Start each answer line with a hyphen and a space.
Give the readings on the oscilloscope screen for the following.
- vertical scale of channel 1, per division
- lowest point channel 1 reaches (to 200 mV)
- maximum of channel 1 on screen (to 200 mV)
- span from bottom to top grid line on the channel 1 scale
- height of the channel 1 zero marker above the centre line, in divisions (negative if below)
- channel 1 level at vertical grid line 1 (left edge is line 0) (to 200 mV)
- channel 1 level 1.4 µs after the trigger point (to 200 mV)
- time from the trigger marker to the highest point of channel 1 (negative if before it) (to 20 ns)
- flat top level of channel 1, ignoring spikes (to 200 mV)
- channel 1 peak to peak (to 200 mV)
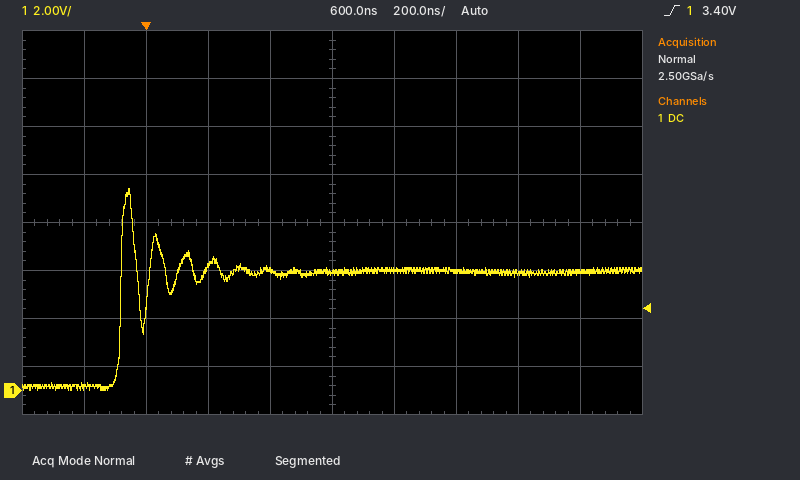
- 2 V
- 0.0 V
- 8.4 V
- 16 V
- -3.5 div
- 200 mV
- 5.0 V
- -60 ns
- 5.0 V
- 8.4 V
